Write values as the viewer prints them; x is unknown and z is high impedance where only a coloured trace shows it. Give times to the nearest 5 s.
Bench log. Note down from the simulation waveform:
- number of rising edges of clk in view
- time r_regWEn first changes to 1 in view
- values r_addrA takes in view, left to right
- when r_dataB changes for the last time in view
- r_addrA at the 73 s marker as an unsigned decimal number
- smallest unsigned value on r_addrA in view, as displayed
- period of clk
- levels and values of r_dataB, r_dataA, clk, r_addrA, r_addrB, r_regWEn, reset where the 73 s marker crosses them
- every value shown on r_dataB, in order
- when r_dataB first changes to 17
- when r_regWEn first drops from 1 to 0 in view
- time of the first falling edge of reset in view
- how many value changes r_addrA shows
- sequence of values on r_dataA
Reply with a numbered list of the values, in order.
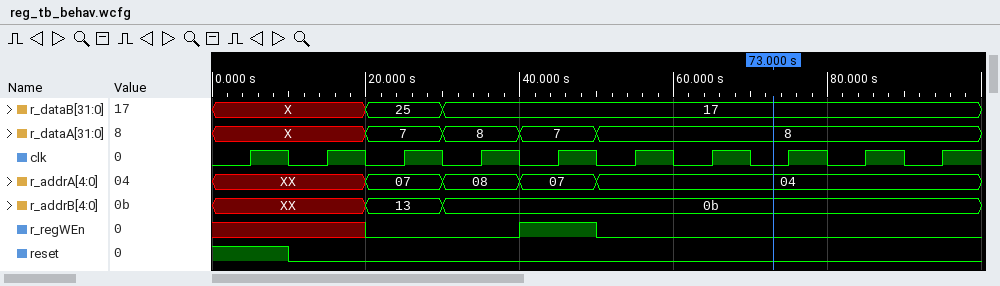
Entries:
1. 10
2. 40 s
3. XX, 07, 08, 07, 04
4. 30 s
5. 4
6. 04
7. 10 s
8. r_dataB=17, r_dataA=8, clk=0, r_addrA=04, r_addrB=0b, r_regWEn=0, reset=0
9. X, 25, 17
10. 30 s
11. 50 s
12. 10 s
13. 4
14. X, 7, 8, 7, 8
